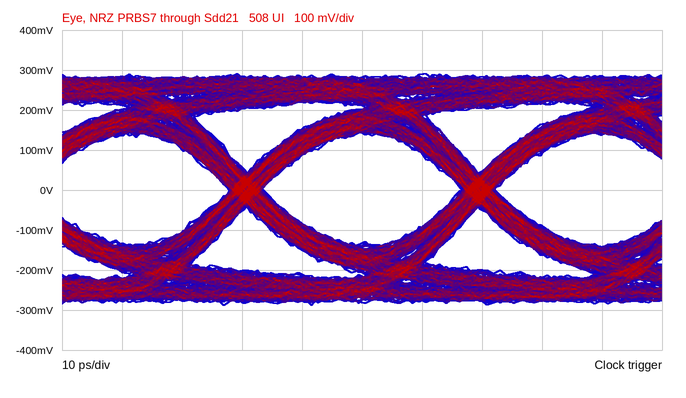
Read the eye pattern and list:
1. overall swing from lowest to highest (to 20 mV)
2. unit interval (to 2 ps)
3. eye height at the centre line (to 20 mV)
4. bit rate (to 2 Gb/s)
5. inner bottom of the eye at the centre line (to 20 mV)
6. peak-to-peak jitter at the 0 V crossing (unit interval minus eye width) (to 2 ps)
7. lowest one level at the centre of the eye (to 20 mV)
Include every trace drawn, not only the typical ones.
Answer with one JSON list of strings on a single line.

["580 mV", "38 ps", "280 mV", "26 Gb/s", "-140 mV", "6 ps", "140 mV"]
